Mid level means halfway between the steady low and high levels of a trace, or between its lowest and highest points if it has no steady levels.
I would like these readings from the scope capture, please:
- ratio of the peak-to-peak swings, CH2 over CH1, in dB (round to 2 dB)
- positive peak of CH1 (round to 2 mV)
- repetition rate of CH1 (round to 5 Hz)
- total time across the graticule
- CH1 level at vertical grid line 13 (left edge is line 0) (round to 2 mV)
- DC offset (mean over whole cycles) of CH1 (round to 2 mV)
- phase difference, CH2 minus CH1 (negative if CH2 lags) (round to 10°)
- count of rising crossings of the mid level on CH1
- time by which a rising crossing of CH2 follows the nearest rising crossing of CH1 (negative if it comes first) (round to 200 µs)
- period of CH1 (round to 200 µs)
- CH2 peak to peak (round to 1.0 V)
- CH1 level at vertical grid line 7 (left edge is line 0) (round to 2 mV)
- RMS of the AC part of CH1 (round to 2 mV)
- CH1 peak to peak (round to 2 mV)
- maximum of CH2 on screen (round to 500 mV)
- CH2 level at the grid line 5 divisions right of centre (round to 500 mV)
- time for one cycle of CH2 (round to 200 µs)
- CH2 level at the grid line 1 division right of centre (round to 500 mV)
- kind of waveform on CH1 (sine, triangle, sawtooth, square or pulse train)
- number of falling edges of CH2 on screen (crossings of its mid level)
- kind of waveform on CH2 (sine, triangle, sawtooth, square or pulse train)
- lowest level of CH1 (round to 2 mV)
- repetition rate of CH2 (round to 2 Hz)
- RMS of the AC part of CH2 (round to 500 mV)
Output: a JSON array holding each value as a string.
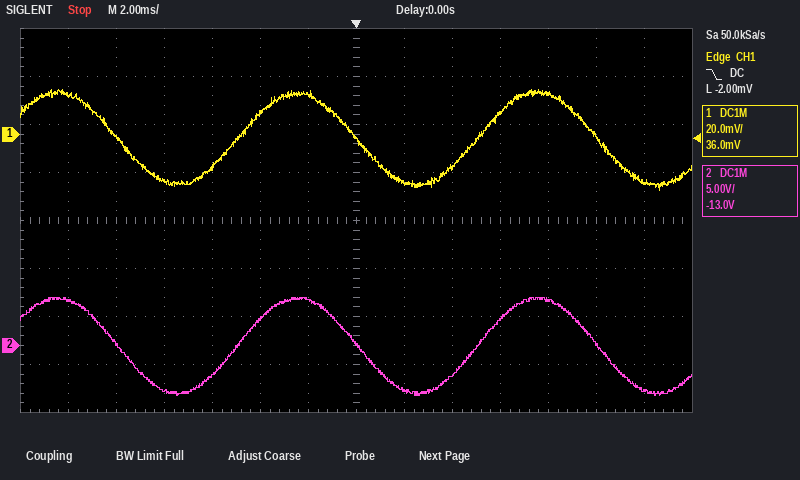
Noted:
["48 dB", "18 mV", "100 Hz", "28 ms", "-20 mV", "-2 mV", "0°", "2", "0.0 ms", "10.0 ms", "10.0 V", "-2 mV", "14 mV", "42 mV", "5.0 V", "0.0 V", "10.0 ms", "-4.5 V", "sine", "3", "sine", "-24 mV", "100 Hz", "3.5 V"]
